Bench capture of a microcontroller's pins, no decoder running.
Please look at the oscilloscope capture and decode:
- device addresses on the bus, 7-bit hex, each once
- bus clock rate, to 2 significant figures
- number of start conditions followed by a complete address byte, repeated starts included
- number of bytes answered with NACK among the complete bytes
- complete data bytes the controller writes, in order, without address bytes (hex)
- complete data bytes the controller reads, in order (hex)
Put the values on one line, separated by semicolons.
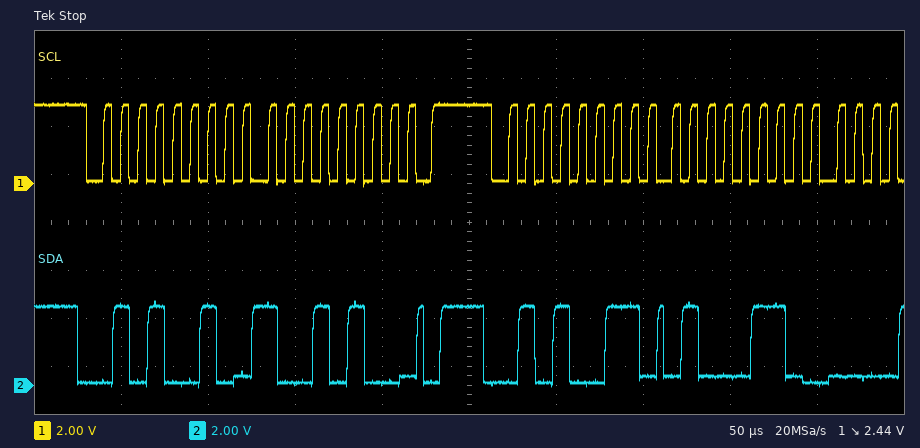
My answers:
0x29; 100 kHz; 2; 0; 94; 46
